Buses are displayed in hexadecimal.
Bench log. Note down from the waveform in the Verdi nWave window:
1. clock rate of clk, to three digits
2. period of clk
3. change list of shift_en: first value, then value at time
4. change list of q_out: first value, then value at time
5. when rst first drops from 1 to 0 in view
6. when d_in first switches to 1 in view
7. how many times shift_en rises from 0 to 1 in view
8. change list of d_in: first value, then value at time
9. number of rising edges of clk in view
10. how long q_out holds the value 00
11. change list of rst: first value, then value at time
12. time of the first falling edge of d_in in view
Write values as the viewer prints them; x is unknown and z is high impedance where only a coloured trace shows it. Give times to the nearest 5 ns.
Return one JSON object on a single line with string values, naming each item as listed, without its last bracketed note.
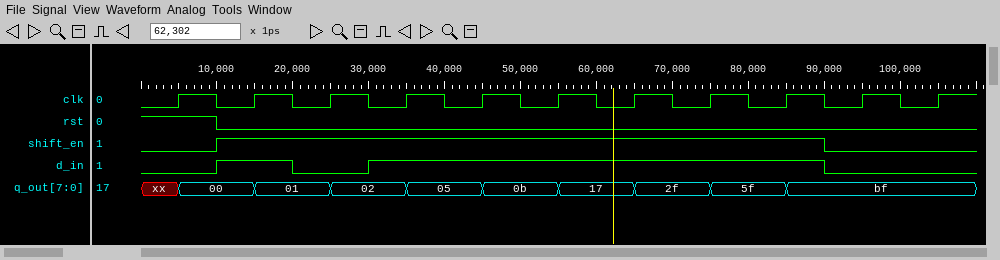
{"clock rate of clk, to three digits": "100 MHz", "period of clk": "10 ns", "change list of shift_en: first value, then value at time": "0, 1 at 10 ns, 0 at 90 ns", "change list of q_out: first value, then value at time": "xx, 00 at 5 ns, 01 at 15 ns, 02 at 25 ns, 05 at 35 ns, 0b at 45 ns, 17 at 55 ns, 2f at 65 ns, 5f at 75 ns, bf at 85 ns", "when rst first drops from 1 to 0 in view": "10 ns", "when d_in first switches to 1 in view": "10 ns", "how many times shift_en rises from 0 to 1 in view": "1", "change list of d_in: first value, then value at time": "0, 1 at 10 ns, 0 at 20 ns, 1 at 30 ns, 0 at 90 ns", "number of rising edges of clk in view": "11", "how long q_out holds the value 00": "10 ns", "change list of rst: first value, then value at time": "1, 0 at 10 ns", "time of the first falling edge of d_in in view": "20 ns"}
